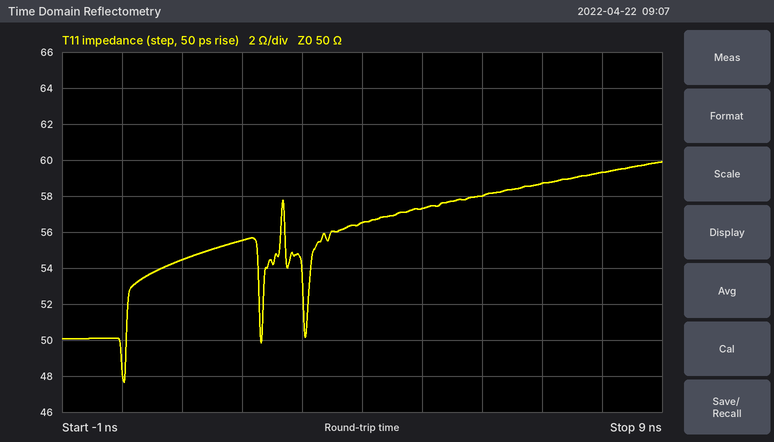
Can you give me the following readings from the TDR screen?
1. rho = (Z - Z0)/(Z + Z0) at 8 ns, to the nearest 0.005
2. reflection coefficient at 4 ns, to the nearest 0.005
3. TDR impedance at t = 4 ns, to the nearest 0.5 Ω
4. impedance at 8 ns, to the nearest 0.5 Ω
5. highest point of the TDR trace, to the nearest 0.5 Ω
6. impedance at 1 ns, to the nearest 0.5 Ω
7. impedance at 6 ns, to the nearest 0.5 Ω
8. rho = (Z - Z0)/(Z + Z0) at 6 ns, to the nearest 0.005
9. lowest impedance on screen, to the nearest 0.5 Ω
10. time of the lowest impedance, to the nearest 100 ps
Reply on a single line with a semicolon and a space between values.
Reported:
+0.085; +0.060; 56.5 Ω; 59.5 Ω; 60.0 Ω; 54.5 Ω; 58.0 Ω; +0.075; 47.5 Ω; 0.0 ns
